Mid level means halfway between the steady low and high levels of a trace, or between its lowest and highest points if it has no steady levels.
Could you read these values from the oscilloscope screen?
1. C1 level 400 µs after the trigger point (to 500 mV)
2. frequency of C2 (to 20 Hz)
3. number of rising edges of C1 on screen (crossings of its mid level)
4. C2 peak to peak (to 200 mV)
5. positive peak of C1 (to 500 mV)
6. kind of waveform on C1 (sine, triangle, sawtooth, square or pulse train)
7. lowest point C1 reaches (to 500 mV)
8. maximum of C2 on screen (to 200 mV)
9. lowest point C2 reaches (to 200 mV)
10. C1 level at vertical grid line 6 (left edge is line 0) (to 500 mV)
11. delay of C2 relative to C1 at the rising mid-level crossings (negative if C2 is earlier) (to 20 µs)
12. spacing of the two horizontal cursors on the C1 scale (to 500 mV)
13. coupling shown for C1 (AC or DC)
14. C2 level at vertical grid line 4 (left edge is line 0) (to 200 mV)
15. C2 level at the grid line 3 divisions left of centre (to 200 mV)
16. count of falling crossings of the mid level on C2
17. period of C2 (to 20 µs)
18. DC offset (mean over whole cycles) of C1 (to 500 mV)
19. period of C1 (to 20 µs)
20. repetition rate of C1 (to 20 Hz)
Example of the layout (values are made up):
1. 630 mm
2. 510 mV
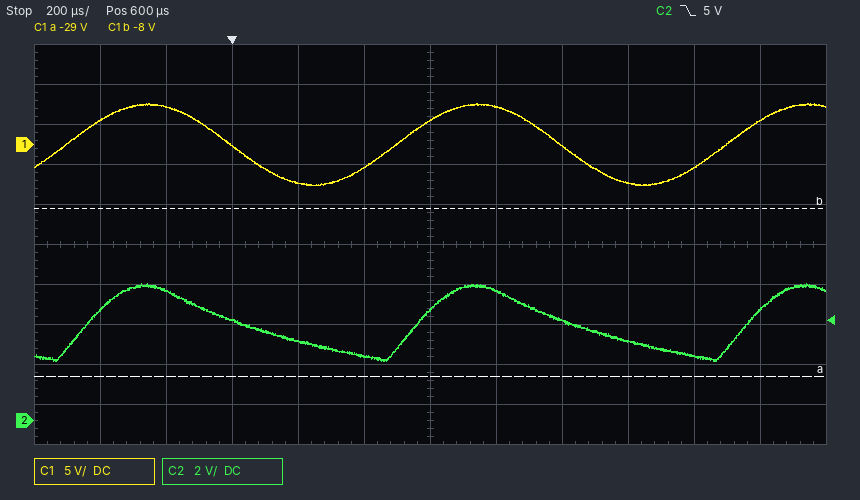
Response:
1. -3.0 V
2. 1.00 kHz
3. 3
4. 3.8 V
5. 5.0 V
6. sine
7. -5.0 V
8. 6.8 V
9. 3.0 V
10. 3.0 V
11. +60 µs
12. 21.0 V
13. DC
14. 4.0 V
15. 5.0 V
16. 2
17. 1.00 ms
18. 0.0 V
19. 1.00 ms
20. 1.00 kHz
